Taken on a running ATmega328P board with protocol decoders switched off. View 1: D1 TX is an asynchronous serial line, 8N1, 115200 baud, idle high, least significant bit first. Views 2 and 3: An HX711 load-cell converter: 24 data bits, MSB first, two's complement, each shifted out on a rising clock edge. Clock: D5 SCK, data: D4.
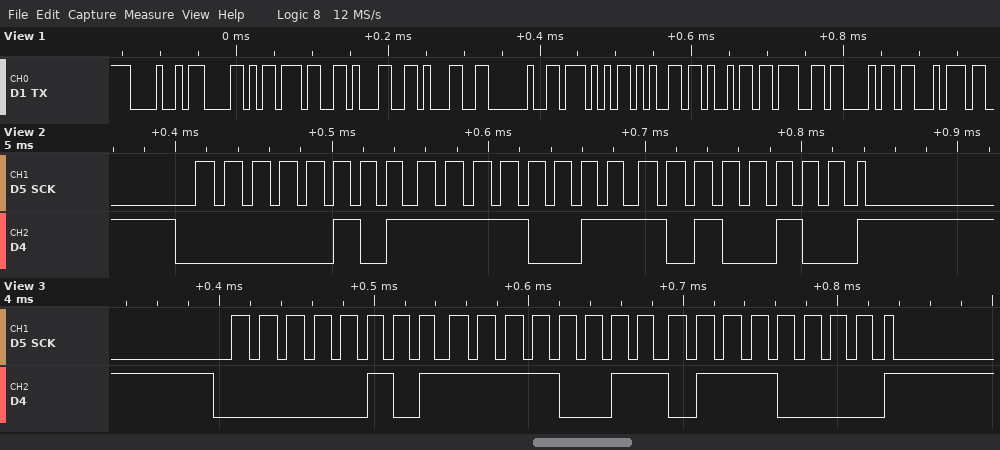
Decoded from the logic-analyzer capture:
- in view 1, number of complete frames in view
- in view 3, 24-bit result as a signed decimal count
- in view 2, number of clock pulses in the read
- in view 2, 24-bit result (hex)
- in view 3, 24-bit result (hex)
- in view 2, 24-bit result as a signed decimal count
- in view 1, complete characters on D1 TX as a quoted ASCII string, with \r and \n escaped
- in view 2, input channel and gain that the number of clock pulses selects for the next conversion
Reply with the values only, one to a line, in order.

12
390000
25
0x05F3A4
0x05F370
390052
"HX711 Weight"
channel A, gain 128
